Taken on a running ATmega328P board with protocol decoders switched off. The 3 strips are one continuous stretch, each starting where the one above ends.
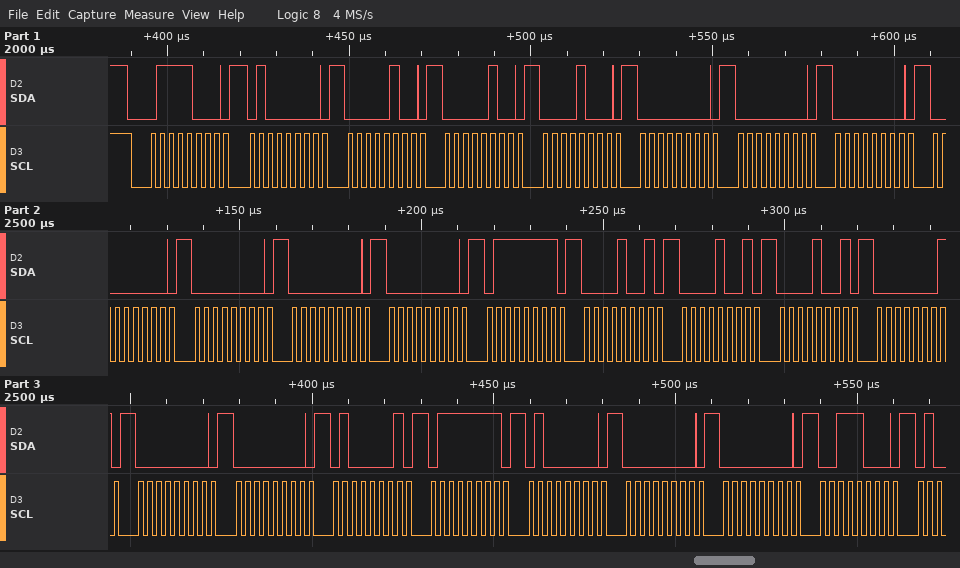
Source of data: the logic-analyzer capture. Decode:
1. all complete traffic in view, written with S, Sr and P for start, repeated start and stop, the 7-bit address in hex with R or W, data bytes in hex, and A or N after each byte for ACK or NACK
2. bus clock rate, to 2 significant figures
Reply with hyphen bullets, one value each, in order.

- S 3CW A 40 A 04 A 04 A 08 A 00 A 00 A 00 A 00 A 00 A 00 A 00 A 7F A 09 A 09 A 09 A 01 A 00 A 00 A 41 A 7F A 40 A 00 A 00 A 38 A
- 400 kHz
